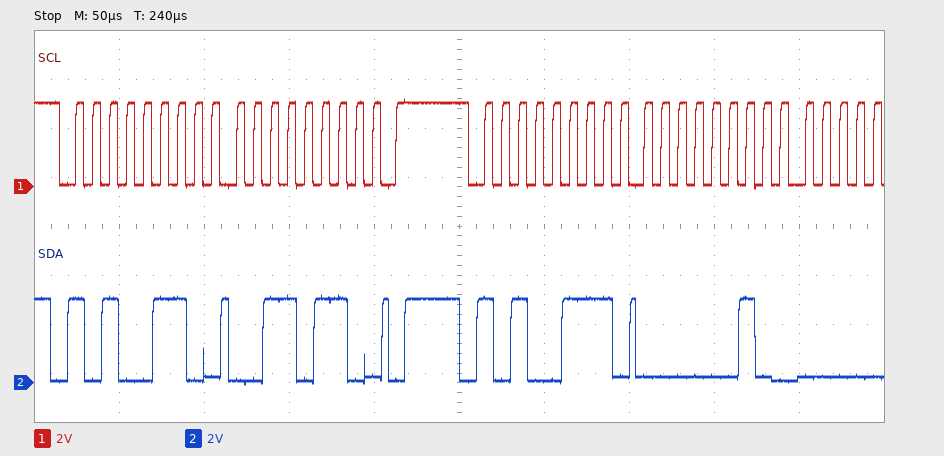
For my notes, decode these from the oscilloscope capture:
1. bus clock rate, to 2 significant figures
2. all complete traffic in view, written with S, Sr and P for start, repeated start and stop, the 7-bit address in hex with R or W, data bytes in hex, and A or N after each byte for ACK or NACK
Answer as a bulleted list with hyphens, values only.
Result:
- 100 kHz
- S 53W A 36 A P S 53R A 02 A
